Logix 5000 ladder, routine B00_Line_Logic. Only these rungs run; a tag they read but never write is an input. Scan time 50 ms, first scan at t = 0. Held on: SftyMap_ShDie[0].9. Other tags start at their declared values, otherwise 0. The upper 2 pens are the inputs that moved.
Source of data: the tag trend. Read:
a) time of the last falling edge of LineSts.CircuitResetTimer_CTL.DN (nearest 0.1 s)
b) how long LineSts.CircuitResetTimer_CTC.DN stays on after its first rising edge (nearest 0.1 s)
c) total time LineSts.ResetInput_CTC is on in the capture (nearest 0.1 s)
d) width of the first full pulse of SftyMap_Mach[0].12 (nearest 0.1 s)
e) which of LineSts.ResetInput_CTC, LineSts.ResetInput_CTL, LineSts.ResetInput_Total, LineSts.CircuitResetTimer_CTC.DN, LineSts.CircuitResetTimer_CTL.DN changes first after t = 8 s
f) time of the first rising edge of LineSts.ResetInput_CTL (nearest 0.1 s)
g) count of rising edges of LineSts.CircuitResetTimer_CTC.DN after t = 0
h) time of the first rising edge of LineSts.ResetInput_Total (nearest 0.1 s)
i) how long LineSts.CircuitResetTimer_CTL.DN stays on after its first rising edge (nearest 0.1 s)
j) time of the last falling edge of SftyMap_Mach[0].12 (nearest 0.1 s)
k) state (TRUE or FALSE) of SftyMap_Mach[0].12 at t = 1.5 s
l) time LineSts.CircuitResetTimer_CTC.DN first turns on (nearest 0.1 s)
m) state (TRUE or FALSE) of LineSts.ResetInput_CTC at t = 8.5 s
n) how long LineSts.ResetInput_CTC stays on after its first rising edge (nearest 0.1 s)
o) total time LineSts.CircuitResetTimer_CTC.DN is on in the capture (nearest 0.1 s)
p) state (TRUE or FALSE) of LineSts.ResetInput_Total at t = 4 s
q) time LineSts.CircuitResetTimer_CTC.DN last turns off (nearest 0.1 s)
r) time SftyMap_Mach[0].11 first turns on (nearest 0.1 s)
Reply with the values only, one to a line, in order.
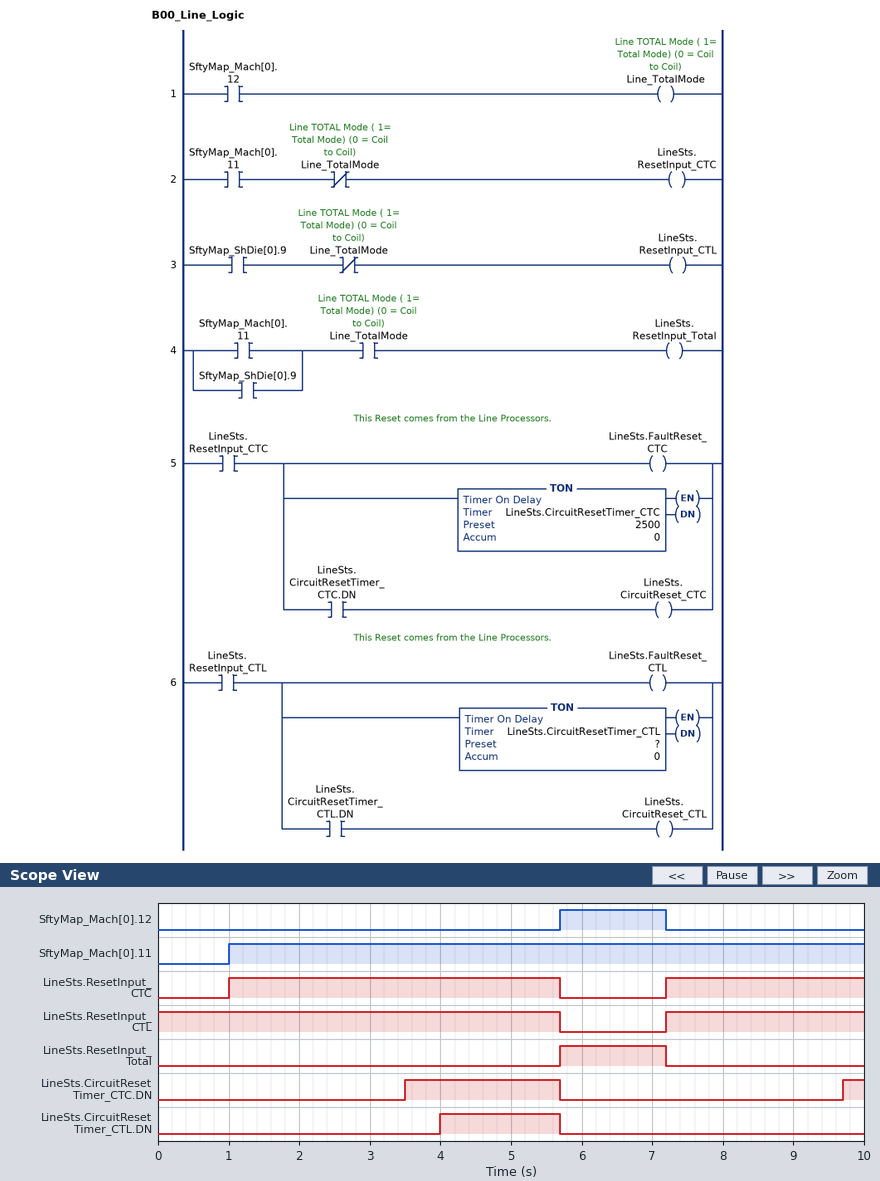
5.7 s
2.2 s
7.5 s
1.5 s
LineSts.CircuitResetTimer_CTC.DN
7.2 s
2
5.7 s
1.7 s
7.2 s
FALSE
3.5 s
TRUE
4.7 s
2.5 s
FALSE
5.7 s
1.0 s
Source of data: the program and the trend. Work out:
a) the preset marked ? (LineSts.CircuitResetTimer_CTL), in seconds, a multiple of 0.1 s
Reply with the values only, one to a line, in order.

4.0 s
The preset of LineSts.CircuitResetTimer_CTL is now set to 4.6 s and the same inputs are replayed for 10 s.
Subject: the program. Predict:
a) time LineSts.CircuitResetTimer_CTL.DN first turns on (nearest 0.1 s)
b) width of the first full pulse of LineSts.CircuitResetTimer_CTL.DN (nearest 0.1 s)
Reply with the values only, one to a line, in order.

4.6 s
1.1 s
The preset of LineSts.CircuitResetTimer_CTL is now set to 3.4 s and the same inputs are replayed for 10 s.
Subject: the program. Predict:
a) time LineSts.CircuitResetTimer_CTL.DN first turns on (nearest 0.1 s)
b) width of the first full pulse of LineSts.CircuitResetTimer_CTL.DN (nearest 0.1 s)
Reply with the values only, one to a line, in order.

3.4 s
2.3 s
